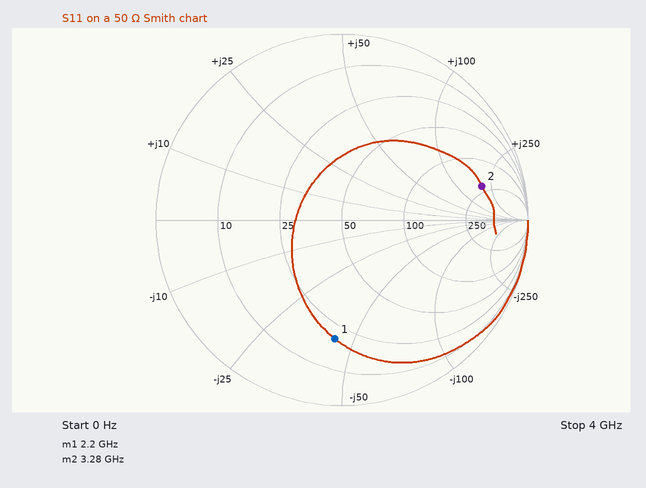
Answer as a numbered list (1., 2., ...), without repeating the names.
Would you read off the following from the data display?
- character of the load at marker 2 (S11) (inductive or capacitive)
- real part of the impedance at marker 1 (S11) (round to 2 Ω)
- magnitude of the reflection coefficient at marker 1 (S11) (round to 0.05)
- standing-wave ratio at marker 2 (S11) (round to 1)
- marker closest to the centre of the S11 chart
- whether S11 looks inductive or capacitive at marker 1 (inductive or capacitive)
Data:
1. inductive
2. 20 Ω
3. 0.65
4. 8
5. marker 1
6. capacitive
